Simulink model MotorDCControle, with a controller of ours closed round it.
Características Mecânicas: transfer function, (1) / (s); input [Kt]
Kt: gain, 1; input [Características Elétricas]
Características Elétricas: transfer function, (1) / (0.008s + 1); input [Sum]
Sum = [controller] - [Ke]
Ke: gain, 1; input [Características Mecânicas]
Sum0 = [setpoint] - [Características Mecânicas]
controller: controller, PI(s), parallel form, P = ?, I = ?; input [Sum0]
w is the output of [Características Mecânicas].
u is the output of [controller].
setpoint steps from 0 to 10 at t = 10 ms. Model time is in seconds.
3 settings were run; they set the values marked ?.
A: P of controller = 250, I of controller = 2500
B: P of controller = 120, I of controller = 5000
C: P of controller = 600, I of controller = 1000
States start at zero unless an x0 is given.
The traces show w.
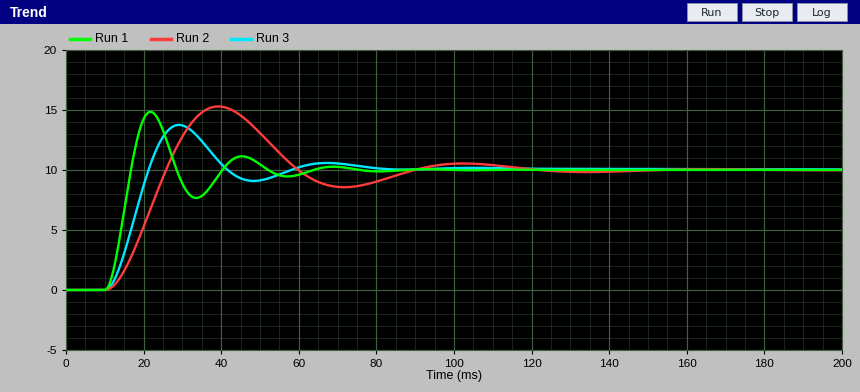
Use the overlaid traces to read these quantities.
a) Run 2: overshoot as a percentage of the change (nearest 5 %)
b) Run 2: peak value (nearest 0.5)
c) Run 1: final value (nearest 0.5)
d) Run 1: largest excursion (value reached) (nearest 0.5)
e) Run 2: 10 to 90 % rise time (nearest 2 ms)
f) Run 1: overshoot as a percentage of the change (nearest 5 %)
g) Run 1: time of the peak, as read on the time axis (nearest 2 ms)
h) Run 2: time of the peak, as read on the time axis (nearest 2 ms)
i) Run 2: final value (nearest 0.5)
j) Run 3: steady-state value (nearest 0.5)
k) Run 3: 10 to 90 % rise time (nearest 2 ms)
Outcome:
55 %
15.5
10.0
15.0
10 ms
50 %
22 ms
40 ms
10.0
10.0
8 ms
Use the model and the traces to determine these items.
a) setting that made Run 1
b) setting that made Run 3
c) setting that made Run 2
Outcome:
C
A
B
